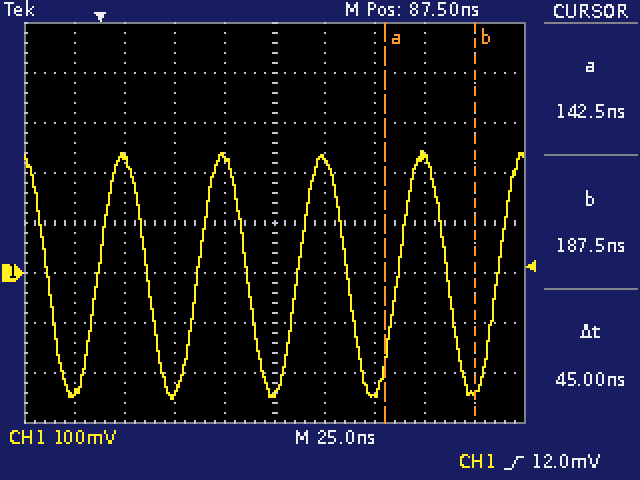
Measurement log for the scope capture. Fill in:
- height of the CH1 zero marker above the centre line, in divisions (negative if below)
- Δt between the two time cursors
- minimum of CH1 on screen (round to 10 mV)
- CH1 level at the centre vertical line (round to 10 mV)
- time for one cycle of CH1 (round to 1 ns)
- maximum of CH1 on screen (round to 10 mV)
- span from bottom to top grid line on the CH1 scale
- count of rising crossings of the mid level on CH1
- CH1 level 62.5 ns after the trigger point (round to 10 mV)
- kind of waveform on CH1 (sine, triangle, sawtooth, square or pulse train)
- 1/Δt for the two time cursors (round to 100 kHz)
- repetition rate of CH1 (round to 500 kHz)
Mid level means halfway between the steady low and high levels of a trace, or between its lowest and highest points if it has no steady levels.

-1.0 div
45 ns
-250 mV
-240 mV
50 ns
240 mV
800 mV
5
230 mV
sine
22.2 MHz
20.0 MHz
